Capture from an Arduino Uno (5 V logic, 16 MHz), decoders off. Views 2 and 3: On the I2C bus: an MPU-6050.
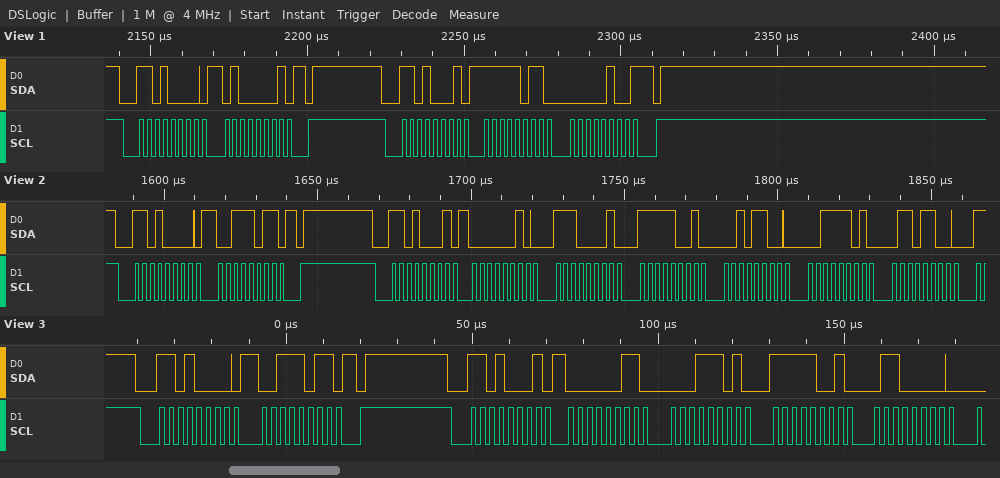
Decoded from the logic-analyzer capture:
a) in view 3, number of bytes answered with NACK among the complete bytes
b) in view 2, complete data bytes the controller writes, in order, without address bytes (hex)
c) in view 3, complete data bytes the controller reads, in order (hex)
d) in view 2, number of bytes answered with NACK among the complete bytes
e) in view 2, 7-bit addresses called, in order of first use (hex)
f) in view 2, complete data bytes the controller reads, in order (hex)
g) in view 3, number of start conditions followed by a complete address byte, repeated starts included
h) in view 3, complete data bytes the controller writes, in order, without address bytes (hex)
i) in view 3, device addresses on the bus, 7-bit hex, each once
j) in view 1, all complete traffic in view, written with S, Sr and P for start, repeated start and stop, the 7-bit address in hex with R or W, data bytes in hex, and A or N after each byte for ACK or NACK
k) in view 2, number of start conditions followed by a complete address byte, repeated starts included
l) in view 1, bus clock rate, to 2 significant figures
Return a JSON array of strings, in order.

["0", "3B", "03 1D F9 60", "0", "0x68", "02 E1 F9 2C 3D 6C", "2", "3B", "0x68", "S 68W A 41 A P S 68R A FB A 04 N P", "2", "400 kHz"]
